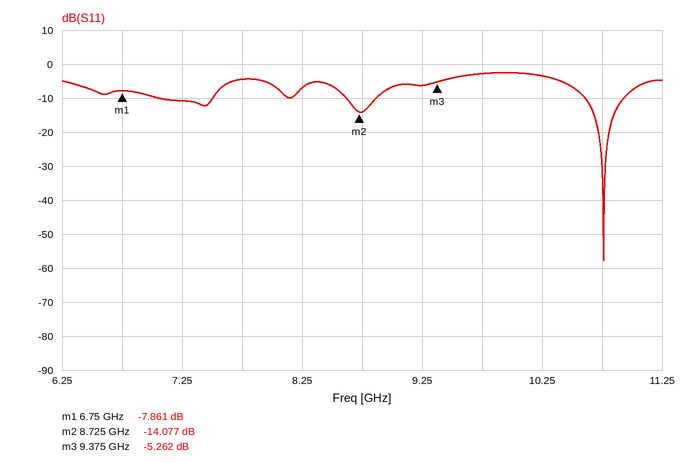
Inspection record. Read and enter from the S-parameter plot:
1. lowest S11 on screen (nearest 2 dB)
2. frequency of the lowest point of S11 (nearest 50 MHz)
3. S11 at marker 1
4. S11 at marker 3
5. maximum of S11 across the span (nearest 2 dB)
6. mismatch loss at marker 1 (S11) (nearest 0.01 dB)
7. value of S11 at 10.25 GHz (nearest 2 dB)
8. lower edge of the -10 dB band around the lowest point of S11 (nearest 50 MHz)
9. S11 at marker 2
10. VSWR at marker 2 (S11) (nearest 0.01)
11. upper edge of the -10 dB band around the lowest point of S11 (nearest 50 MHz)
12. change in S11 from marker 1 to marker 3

-58 dB
10.75 GHz
-7.861 dB
-5.262 dB
-2 dB
0.78 dB
-4 dB
10.60 GHz
-14.077 dB
1.49
10.95 GHz
2.599 dB
